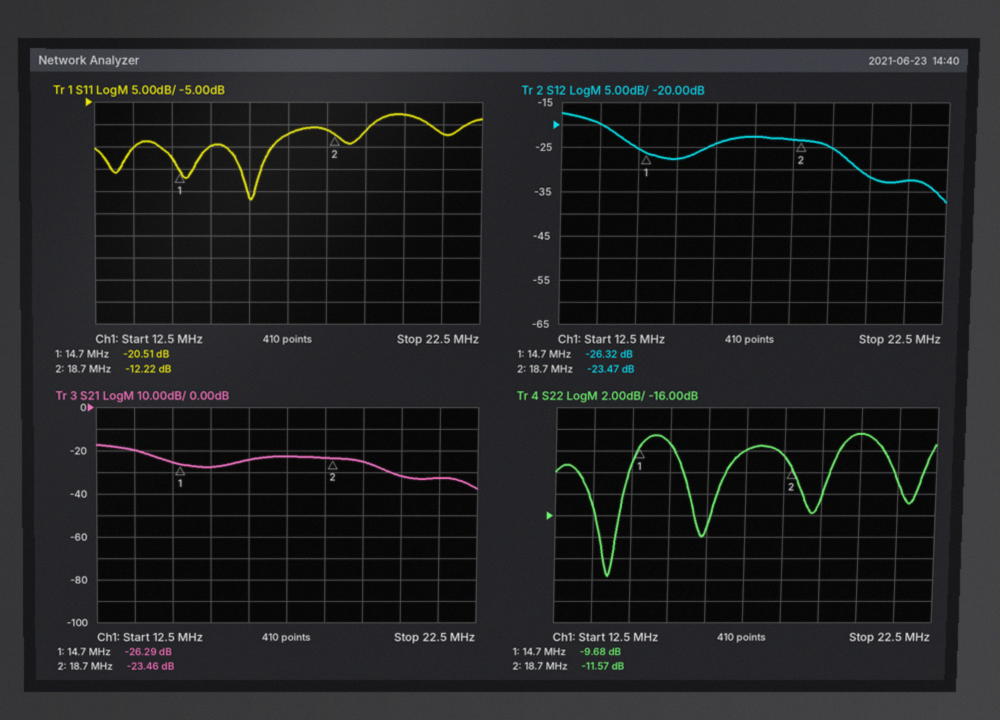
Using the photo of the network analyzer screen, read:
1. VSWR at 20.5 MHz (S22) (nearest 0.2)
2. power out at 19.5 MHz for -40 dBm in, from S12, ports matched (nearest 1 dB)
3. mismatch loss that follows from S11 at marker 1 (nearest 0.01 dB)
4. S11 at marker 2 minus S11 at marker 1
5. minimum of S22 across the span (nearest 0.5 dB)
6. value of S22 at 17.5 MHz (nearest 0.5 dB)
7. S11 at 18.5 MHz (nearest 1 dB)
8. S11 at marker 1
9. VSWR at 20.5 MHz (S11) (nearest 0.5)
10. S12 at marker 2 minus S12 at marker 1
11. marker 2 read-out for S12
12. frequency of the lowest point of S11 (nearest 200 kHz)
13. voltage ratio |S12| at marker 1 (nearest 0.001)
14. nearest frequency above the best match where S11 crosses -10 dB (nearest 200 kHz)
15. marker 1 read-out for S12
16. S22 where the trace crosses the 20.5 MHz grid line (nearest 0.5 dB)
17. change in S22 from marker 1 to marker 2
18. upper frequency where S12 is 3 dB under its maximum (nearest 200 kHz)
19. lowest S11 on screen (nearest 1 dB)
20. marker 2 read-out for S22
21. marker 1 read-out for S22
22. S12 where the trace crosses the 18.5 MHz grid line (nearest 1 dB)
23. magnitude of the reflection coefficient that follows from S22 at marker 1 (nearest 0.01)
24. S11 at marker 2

2.2
-65 dBm
0.04 dB
8.29 dB
-21.5 dB
-10.0 dB
-11 dB
-20.51 dB
2.5
2.85 dB
-23.47 dB
16.6 MHz
0.048
19.6 MHz
-26.32 dB
-8.5 dB
-1.89 dB
13.6 MHz
-27 dB
-11.57 dB
-9.68 dB
-23 dB
0.33
-12.22 dB
